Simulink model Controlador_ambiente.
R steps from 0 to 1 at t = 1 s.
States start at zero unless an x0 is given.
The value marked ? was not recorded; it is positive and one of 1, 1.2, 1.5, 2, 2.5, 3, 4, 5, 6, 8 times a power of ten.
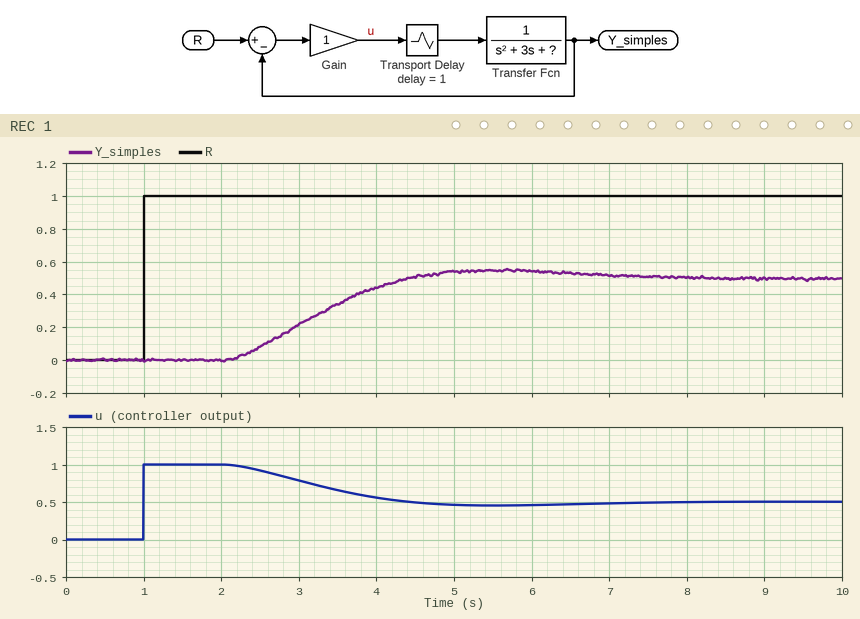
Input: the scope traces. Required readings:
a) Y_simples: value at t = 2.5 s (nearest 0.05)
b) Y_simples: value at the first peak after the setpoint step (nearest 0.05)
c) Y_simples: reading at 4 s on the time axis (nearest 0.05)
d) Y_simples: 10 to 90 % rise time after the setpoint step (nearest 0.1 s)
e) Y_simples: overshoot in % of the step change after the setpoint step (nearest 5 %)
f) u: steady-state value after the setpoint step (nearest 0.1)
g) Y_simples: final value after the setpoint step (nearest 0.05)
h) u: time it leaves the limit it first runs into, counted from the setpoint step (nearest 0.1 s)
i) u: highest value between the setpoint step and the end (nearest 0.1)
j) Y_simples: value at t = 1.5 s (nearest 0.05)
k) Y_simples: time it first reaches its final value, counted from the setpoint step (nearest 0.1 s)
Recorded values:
0.10
0.55
0.45
1.7 s
10 %
0.5
0.50
1.2 s
1.0
0.00
3.4 s
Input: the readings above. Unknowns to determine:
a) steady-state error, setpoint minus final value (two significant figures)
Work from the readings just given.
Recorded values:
0.50
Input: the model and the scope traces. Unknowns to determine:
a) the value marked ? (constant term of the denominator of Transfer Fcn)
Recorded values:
1
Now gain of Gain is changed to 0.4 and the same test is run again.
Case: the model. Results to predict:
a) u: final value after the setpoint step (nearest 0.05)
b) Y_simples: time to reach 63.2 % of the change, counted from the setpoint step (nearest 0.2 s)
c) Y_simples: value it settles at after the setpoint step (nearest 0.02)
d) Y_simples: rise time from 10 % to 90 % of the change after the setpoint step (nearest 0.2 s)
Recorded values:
0.30
3.0 s
0.28
3.2 s
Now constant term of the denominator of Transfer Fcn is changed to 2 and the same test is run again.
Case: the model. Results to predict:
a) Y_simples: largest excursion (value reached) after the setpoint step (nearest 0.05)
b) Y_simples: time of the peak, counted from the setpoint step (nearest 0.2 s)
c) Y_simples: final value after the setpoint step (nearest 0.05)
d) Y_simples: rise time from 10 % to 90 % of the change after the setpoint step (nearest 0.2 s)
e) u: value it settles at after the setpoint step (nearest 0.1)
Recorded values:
0.40
3.6 s
0.35
1.2 s
0.7
